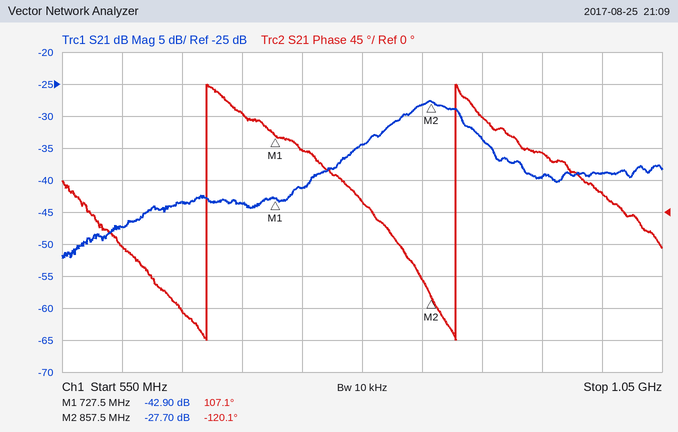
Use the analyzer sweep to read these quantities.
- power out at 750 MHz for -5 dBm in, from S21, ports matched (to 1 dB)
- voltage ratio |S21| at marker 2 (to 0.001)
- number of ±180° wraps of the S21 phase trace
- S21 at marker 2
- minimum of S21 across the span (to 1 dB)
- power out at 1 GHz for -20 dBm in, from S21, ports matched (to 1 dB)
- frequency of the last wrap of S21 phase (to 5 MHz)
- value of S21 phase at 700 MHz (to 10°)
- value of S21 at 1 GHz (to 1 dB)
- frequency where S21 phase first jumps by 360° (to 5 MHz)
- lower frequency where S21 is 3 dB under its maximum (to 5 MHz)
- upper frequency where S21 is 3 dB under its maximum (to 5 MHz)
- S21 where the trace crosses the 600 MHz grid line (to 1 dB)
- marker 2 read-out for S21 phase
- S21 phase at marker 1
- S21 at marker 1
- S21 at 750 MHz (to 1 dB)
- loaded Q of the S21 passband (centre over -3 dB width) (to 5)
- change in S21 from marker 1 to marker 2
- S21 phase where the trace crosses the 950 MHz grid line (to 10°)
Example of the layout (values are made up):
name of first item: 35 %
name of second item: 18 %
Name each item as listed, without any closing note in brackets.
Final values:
power out at 750 MHz for -5 dBm in, from S21, ports matched: -46 dBm
voltage ratio |S21| at marker 2: 0.041
number of ±180° wraps of the S21 phase trace: 2
S21 at marker 2: -27.70 dB
minimum of S21 across the span: -52 dB
power out at 1 GHz for -20 dBm in, from S21, ports matched: -59 dBm
frequency of the last wrap of S21 phase: 880 MHz
value of S21 phase at 700 MHz: 140°
value of S21 at 1 GHz: -39 dB
frequency where S21 phase first jumps by 360°: 670 MHz
lower frequency where S21 is 3 dB under its maximum: 830 MHz
upper frequency where S21 is 3 dB under its maximum: 885 MHz
S21 where the trace crosses the 600 MHz grid line: -47 dB
marker 2 read-out for S21 phase: -120.1°
S21 phase at marker 1: 107.1°
S21 at marker 1: -42.90 dB
S21 at 750 MHz: -41 dB
loaded Q of the S21 passband (centre over -3 dB width): 15
change in S21 from marker 1 to marker 2: 15.20 dB
S21 phase where the trace crosses the 950 MHz grid line: 80°
